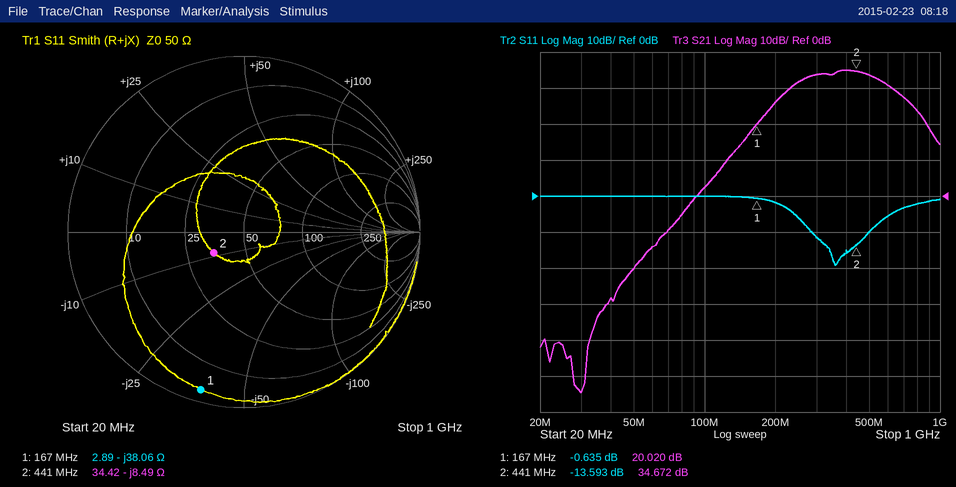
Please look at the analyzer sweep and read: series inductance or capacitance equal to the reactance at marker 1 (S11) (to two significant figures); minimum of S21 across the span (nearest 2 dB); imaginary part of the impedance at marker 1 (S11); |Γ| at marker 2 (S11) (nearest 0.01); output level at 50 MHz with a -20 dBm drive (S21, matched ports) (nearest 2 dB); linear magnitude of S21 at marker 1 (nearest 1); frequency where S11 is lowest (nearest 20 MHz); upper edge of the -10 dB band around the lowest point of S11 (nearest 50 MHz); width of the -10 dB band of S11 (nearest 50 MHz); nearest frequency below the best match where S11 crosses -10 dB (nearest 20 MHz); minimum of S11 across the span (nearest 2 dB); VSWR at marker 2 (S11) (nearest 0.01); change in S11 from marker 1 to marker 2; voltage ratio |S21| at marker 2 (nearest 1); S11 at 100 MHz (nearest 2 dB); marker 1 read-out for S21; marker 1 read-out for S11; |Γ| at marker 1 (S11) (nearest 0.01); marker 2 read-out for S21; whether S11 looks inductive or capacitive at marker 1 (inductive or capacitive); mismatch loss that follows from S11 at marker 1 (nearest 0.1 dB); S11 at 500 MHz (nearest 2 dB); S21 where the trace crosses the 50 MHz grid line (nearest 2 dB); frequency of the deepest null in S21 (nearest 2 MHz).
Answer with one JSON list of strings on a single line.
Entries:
["25 pF", "-54 dB", "-38.06 Ω", "0.21", "-40 dBm", "10", "360 MHz", "500 MHz", "200 MHz", "280 MHz", "-20 dB", "1.53", "-12.958 dB", "54", "0 dB", "20.020 dB", "-0.635 dB", "0.93", "34.672 dB", "capacitive", "8.7 dB", "-10 dB", "-20 dB", "30 MHz"]
